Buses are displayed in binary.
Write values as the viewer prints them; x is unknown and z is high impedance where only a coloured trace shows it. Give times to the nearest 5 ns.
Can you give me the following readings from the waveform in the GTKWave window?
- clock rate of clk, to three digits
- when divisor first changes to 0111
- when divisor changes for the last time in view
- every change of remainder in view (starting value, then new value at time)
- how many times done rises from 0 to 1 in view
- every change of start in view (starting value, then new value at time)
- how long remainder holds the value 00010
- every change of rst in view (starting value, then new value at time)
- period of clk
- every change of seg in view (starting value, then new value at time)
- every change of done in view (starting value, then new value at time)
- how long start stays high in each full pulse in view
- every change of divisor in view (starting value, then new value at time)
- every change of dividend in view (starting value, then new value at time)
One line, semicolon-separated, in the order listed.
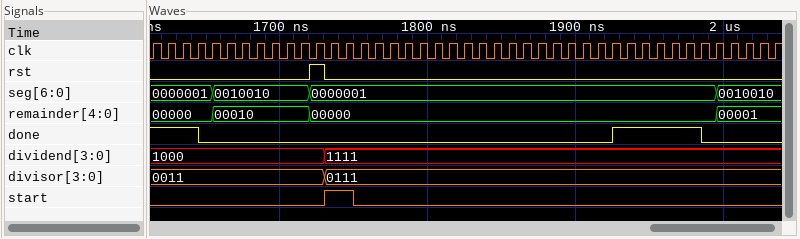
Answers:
100 MHz; 1730 ns; 1730 ns; 00000, 00010 at 1655 ns, 00000 at 1720 ns, 00001 at 1995 ns; 1; 0, 1 at 1730 ns, 0 at 1750 ns; 65 ns; 0, 1 at 1720 ns, 0 at 1730 ns; 10 ns; 0000001, 0010010 at 1655 ns, 0000001 at 1720 ns, 0010010 at 1995 ns; 1, 0 at 1645 ns, 1 at 1925 ns, 0 at 1985 ns; 20 ns; 0011, 0111 at 1730 ns; 1000, 1111 at 1730 ns
